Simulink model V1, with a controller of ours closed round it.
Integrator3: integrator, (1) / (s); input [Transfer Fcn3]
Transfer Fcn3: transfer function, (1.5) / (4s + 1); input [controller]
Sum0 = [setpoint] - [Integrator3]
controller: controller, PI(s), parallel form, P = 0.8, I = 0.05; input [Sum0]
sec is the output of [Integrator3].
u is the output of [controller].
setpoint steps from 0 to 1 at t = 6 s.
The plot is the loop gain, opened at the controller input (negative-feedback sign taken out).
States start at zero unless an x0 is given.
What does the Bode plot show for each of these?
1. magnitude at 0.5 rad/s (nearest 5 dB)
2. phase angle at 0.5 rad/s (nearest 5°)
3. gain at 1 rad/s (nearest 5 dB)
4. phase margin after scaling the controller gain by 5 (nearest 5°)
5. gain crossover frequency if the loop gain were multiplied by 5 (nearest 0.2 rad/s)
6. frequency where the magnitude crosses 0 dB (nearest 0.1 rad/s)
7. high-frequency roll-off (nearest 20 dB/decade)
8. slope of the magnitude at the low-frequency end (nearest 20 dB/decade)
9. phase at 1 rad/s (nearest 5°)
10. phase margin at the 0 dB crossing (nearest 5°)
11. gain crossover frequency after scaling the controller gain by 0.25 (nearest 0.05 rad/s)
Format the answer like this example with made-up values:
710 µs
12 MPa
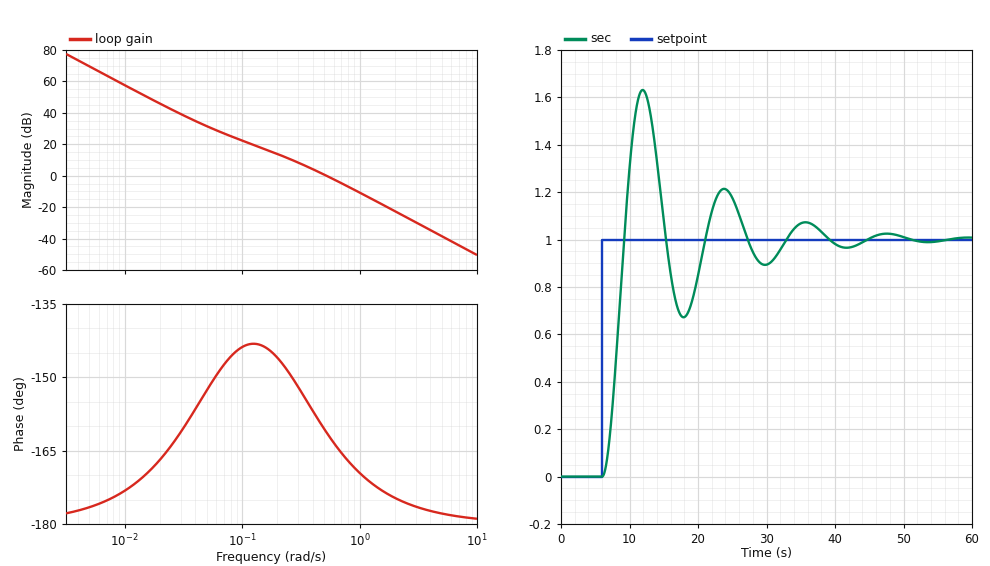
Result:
0 dB
-160°
-10 dB
10°
1.2 rad/s
0.5 rad/s
-40 dB/decade
-40 dB/decade
-170°
20°
0.25 rad/s
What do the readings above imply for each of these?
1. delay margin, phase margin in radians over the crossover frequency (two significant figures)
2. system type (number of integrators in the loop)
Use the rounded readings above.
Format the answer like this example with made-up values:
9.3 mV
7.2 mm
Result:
0.70 s
2
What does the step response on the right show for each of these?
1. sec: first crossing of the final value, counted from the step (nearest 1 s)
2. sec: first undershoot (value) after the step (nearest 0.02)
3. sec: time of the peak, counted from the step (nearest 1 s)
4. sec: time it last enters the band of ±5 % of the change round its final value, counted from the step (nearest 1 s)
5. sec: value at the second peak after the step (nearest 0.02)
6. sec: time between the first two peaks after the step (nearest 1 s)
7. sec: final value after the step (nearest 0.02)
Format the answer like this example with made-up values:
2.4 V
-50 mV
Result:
3 s
0.68
6 s
31 s
1.22
12 s
1.00
